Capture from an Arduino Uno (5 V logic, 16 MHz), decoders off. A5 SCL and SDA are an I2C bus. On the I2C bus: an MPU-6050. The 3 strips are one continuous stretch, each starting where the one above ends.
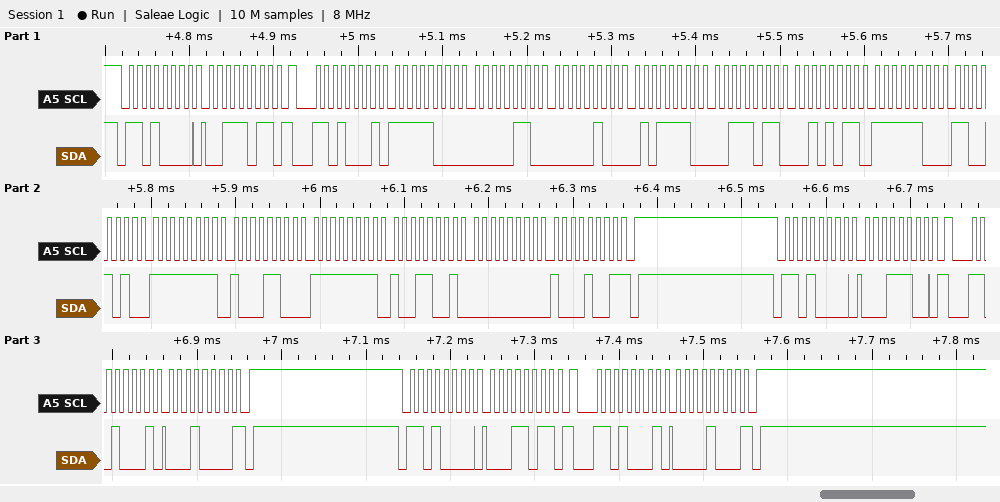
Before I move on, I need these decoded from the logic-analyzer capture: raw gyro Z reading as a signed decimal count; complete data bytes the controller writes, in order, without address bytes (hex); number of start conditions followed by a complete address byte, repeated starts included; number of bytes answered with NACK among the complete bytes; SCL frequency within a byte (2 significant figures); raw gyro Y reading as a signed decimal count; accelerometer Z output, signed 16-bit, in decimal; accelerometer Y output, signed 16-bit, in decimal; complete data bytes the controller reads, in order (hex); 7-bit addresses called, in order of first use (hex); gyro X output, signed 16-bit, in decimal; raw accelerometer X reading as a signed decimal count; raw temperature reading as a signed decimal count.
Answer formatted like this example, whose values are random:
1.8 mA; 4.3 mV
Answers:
137; 3B 1C 1B; 6; 3; 100 kHz; -103; 15147; 1118; F8 06 04 5E 3B 2B FC CA FF 8C FF 99 00 89 10 08; 0x68; -116; -2042; -822
